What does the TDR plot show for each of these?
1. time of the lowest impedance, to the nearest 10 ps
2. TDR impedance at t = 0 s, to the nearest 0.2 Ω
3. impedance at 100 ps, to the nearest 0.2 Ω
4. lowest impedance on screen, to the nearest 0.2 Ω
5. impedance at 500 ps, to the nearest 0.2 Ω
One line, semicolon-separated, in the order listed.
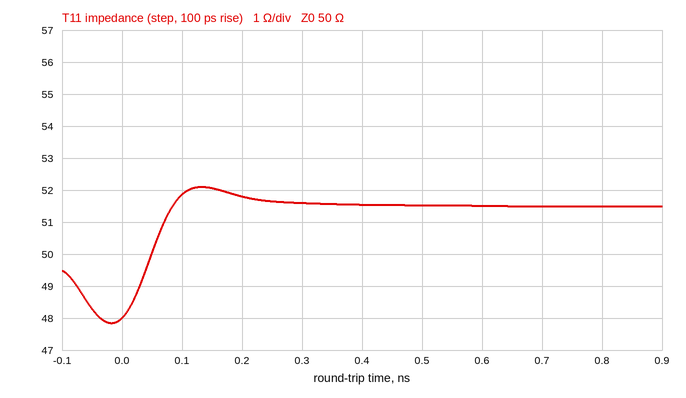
-20 ps; 48.0 Ω; 51.8 Ω; 47.8 Ω; 51.6 Ω
